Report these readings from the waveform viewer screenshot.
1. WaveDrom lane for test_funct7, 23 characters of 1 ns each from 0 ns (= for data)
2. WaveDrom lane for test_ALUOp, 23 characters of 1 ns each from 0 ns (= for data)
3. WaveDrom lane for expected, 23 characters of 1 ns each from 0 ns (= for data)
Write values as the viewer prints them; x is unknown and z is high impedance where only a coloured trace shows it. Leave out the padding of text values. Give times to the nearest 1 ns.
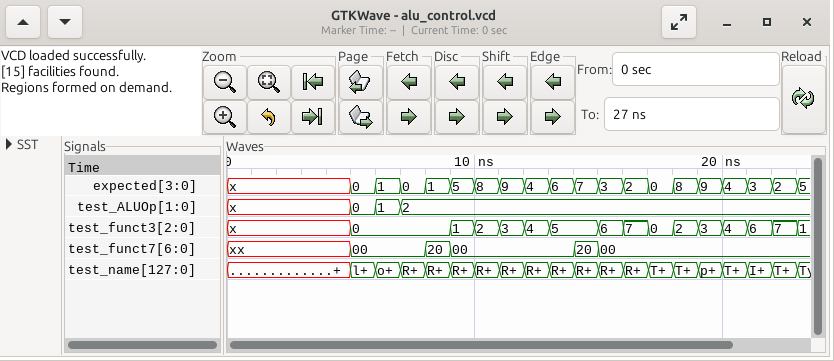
{name: 'test_funct7', wave: 'x....=..==....==.......', data: '00 20 00 20 00'}
{name: 'test_ALUOp', wave: 'x....===...............', data: '0 1 2'}
{name: 'expected', wave: 'x....==================', data: '0 1 0 1 5 8 9 4 6 7 3 2 0 8 9 4 3 2'}
